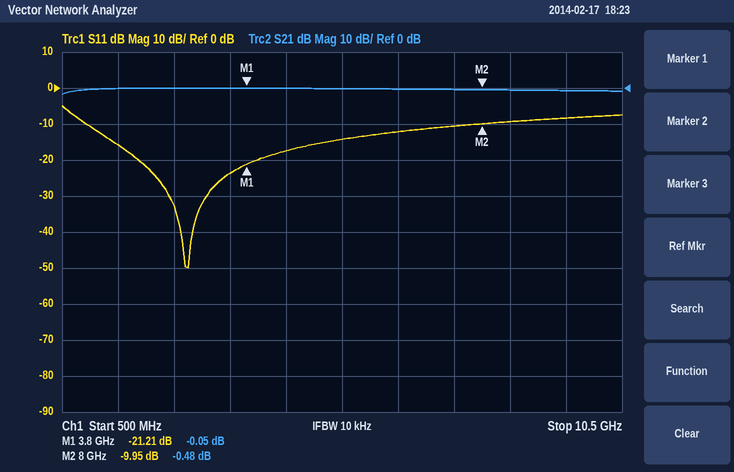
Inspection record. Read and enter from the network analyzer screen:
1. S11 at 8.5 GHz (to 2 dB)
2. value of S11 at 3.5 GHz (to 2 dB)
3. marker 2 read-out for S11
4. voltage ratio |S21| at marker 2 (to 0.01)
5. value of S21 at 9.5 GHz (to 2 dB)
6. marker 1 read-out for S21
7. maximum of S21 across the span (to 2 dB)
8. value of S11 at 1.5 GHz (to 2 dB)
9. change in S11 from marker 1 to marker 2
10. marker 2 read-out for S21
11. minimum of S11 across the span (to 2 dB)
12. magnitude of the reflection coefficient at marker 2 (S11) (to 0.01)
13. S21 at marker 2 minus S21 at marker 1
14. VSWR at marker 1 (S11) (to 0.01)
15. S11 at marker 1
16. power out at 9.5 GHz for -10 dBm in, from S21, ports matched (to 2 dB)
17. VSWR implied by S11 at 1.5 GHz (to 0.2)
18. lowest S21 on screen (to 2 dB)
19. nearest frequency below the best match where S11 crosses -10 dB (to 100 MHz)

-10 dB
-24 dB
-9.95 dB
0.95
0 dB
-0.05 dB
0 dB
-16 dB
11.26 dB
-0.48 dB
-50 dB
0.32
-0.43 dB
1.19
-21.21 dB
-10 dBm
1.4
-2 dB
900 MHz
